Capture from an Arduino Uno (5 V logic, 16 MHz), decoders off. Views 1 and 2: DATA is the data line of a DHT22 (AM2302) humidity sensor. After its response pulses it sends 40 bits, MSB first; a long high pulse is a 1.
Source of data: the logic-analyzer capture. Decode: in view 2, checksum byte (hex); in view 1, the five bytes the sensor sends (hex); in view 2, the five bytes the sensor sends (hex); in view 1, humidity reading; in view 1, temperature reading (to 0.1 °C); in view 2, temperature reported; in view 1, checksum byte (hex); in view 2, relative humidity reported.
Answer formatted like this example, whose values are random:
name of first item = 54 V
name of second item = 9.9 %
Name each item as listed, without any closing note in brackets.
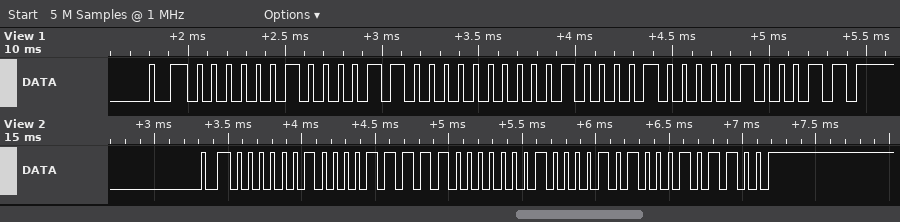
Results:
in view 2, checksum byte = 0x2C
in view 1, the five bytes the sensor sends = 02 18 01 08 23
in view 2, the five bytes the sensor sends = 02 1F 01 0A 2C
in view 1, humidity reading = 53.6 %
in view 1, temperature reading = 26.4 °C
in view 2, temperature reported = 26.6 °C
in view 1, checksum byte = 0x23
in view 2, relative humidity reported = 54.3 %
